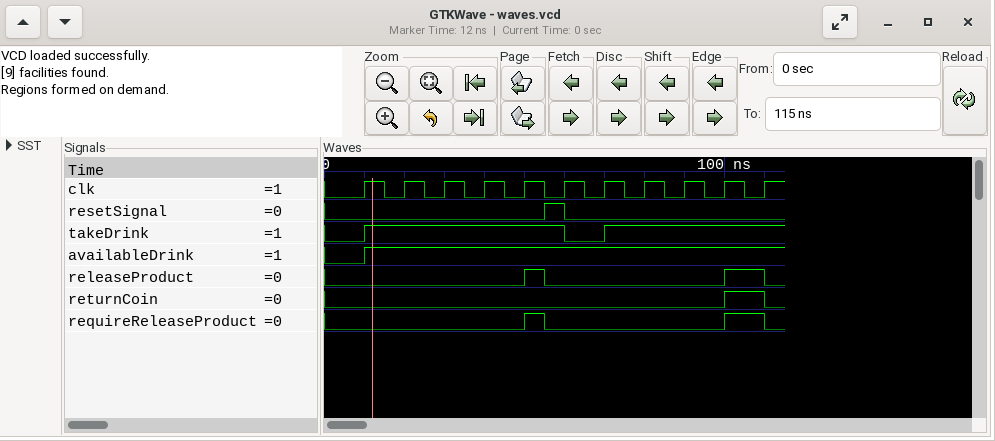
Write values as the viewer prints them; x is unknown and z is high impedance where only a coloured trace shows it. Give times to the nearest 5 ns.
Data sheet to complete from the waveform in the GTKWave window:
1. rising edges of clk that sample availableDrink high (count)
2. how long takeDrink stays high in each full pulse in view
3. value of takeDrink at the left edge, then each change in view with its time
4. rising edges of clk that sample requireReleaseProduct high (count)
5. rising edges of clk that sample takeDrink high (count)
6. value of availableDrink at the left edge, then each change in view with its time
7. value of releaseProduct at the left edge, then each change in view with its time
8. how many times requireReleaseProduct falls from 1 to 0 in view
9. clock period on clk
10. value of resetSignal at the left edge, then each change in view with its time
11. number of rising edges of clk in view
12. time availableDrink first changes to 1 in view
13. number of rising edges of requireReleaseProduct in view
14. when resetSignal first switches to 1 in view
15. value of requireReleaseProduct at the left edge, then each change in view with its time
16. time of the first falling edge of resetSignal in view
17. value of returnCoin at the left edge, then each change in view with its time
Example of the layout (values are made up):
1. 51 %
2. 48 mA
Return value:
1. 10
2. 50 ns
3. 0, 1 at 10 ns, 0 at 60 ns, 1 at 70 ns
4. 1
5. 9
6. 0, 1 at 10 ns
7. 0, 1 at 50 ns, 0 at 55 ns, 1 at 100 ns, 0 at 110 ns
8. 2
9. 10 ns
10. 0, 1 at 55 ns, 0 at 60 ns
11. 11
12. 10 ns
13. 2
14. 55 ns
15. 0, 1 at 50 ns, 0 at 55 ns, 1 at 100 ns, 0 at 110 ns
16. 60 ns
17. 0, 1 at 100 ns, 0 at 110 ns
